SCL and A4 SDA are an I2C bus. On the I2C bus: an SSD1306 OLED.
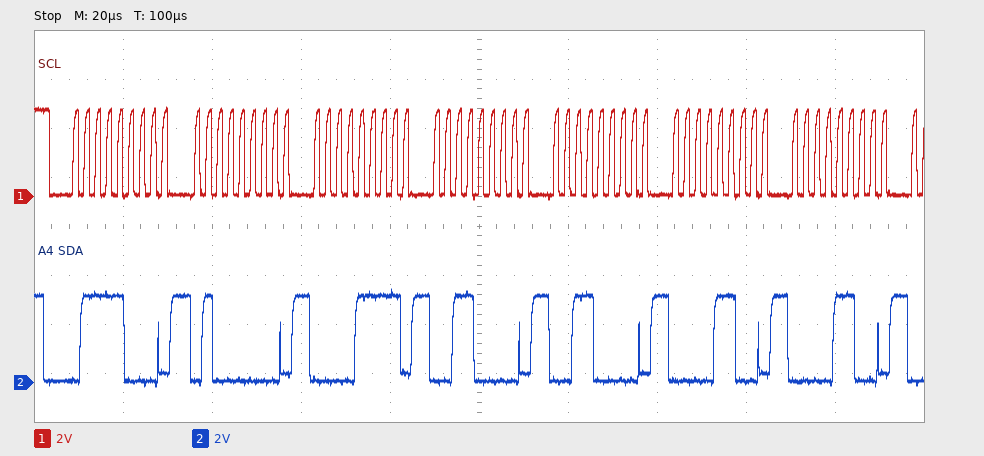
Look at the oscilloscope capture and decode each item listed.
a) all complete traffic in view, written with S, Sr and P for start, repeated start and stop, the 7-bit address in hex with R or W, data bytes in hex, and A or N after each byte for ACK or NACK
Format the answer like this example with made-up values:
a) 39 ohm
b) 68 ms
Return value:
a) S 3CW A 40 A 0F A 30 A 30 A 0C A 0C A
